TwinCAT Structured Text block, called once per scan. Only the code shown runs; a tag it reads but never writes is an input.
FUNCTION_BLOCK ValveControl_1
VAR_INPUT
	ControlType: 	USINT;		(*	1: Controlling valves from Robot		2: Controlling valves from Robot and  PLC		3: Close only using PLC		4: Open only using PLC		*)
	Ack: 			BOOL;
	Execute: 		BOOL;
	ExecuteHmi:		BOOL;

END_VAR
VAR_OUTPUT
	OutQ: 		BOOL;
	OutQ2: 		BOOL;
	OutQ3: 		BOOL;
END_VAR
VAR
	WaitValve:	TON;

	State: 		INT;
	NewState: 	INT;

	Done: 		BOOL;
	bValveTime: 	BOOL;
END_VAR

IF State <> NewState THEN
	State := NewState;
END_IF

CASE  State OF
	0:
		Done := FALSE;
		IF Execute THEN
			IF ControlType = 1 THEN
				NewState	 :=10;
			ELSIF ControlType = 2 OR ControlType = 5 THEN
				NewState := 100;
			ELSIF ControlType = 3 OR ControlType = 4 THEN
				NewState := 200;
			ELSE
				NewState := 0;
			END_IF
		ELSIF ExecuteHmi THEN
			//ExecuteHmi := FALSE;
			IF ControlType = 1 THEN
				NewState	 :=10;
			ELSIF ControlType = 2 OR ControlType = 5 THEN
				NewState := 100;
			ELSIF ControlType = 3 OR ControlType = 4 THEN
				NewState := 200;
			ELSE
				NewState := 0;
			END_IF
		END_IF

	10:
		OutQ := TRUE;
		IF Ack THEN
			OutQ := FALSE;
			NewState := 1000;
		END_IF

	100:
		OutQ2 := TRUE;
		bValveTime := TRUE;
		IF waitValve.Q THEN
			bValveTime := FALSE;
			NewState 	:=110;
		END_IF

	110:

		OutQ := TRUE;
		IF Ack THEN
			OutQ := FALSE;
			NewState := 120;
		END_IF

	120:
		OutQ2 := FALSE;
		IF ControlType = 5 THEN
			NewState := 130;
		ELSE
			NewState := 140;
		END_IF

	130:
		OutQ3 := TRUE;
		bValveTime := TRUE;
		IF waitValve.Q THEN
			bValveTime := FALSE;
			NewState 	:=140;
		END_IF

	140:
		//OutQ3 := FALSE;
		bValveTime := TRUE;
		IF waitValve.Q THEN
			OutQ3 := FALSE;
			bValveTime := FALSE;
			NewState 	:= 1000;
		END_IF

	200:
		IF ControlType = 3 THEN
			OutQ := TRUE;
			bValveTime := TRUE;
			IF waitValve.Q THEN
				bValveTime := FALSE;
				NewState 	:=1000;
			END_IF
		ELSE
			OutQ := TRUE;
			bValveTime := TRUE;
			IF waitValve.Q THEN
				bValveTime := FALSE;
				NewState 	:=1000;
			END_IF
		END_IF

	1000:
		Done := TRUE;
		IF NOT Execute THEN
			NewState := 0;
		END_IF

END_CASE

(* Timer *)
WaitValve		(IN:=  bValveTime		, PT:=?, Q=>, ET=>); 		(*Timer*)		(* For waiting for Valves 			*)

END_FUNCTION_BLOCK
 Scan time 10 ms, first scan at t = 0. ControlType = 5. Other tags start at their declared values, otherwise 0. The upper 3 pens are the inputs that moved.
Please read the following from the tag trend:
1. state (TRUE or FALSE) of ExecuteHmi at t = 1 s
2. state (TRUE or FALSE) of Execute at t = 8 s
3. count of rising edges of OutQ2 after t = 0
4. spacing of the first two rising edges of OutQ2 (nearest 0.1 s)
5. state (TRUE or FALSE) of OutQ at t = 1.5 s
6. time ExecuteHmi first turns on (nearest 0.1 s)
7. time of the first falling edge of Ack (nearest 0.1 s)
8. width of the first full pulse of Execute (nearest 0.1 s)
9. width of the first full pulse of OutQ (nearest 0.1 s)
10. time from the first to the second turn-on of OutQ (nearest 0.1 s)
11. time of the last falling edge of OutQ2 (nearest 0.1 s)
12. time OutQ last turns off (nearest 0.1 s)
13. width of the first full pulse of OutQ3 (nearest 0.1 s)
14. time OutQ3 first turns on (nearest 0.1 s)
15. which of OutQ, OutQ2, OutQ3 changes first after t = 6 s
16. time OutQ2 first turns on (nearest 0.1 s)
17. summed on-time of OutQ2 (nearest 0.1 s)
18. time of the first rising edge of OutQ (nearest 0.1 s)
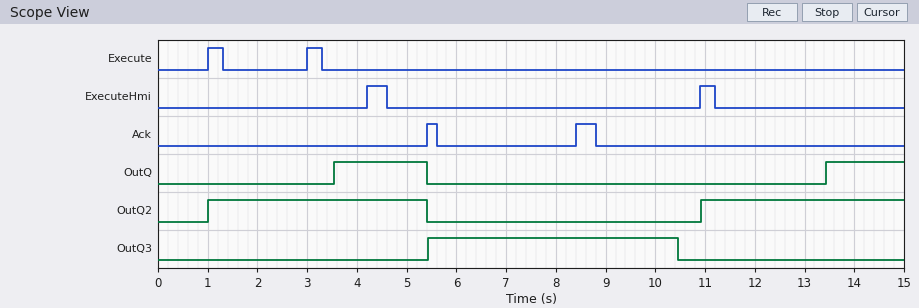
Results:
FALSE
FALSE
2
9.9 s
FALSE
4.2 s
5.6 s
0.3 s
1.9 s
9.9 s
5.4 s
5.4 s
5.0 s
5.4 s
OutQ3
1.0 s
8.5 s
3.5 s
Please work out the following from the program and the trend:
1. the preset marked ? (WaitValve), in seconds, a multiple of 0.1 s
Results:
2.5 s
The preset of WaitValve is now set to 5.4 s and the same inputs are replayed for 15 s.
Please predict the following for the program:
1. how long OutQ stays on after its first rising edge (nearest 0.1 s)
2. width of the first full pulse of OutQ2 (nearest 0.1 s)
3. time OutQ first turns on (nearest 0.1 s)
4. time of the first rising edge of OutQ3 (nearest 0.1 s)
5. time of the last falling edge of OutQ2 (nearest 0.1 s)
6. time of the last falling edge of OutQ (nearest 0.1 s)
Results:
2.0 s
7.4 s
6.4 s
8.4 s
8.4 s
8.4 s
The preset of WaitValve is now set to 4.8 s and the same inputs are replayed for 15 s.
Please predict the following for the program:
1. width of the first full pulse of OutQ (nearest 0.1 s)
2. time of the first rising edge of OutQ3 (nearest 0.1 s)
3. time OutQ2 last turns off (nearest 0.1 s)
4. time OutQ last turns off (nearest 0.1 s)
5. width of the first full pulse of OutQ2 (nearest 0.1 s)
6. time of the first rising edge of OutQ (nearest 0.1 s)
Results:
2.6 s
8.4 s
8.4 s
8.4 s
7.4 s
5.8 s
